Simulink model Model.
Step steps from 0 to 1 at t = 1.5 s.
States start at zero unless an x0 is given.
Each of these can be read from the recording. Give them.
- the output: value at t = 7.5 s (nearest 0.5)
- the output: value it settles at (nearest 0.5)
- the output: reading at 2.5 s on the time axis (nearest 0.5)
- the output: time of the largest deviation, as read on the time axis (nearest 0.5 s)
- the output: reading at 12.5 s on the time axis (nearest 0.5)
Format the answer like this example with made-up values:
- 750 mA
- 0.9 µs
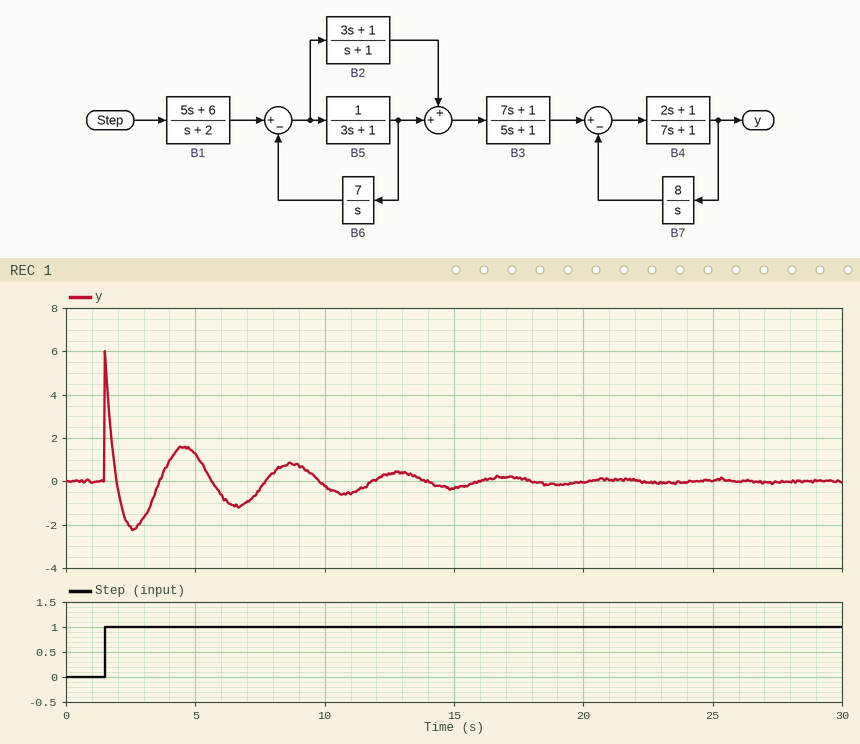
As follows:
- -0.5
- 0.0
- -2.0
- 1.5 s
- 0.5
